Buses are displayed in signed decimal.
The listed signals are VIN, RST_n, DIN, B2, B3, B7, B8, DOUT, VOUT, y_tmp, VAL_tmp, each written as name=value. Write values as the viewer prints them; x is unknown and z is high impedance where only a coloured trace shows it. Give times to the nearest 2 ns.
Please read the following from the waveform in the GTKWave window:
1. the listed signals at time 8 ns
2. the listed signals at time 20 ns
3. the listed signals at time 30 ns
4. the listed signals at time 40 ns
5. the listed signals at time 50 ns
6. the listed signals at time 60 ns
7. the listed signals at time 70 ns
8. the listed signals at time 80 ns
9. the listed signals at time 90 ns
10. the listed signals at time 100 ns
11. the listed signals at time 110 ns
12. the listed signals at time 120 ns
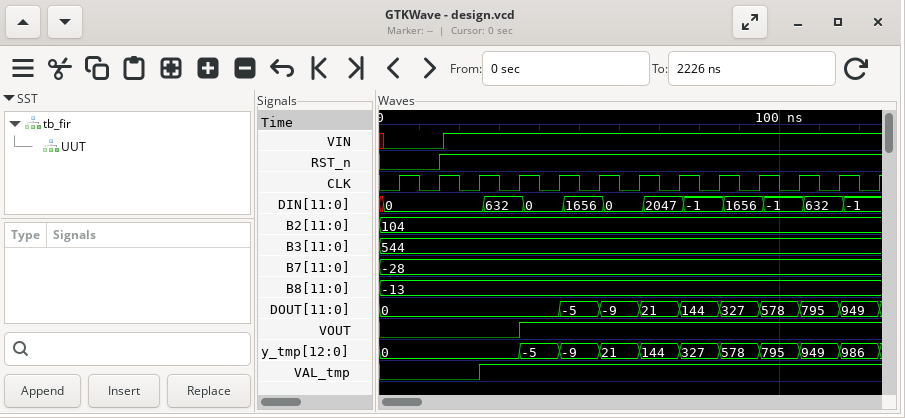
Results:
VIN=0, RST_n=0, DIN=0, B2=104, B3=544, B7=-28, B8=-13, DOUT=0, VOUT=0, y_tmp=0, VAL_tmp=0
VIN=1, RST_n=1, DIN=0, B2=104, B3=544, B7=-28, B8=-13, DOUT=0, VOUT=0, y_tmp=0, VAL_tmp=0
VIN=1, RST_n=1, DIN=632, B2=104, B3=544, B7=-28, B8=-13, DOUT=0, VOUT=0, y_tmp=0, VAL_tmp=1
VIN=1, RST_n=1, DIN=0, B2=104, B3=544, B7=-28, B8=-13, DOUT=0, VOUT=1, y_tmp=-5, VAL_tmp=1
VIN=1, RST_n=1, DIN=1656, B2=104, B3=544, B7=-28, B8=-13, DOUT=-5, VOUT=1, y_tmp=-9, VAL_tmp=1
VIN=1, RST_n=1, DIN=0, B2=104, B3=544, B7=-28, B8=-13, DOUT=-9, VOUT=1, y_tmp=21, VAL_tmp=1
VIN=1, RST_n=1, DIN=2047, B2=104, B3=544, B7=-28, B8=-13, DOUT=21, VOUT=1, y_tmp=144, VAL_tmp=1
VIN=1, RST_n=1, DIN=-1, B2=104, B3=544, B7=-28, B8=-13, DOUT=144, VOUT=1, y_tmp=327, VAL_tmp=1
VIN=1, RST_n=1, DIN=1656, B2=104, B3=544, B7=-28, B8=-13, DOUT=327, VOUT=1, y_tmp=578, VAL_tmp=1
VIN=1, RST_n=1, DIN=-1, B2=104, B3=544, B7=-28, B8=-13, DOUT=578, VOUT=1, y_tmp=795, VAL_tmp=1
VIN=1, RST_n=1, DIN=632, B2=104, B3=544, B7=-28, B8=-13, DOUT=795, VOUT=1, y_tmp=949, VAL_tmp=1
VIN=1, RST_n=1, DIN=-1, B2=104, B3=544, B7=-28, B8=-13, DOUT=949, VOUT=1, y_tmp=986, VAL_tmp=1
